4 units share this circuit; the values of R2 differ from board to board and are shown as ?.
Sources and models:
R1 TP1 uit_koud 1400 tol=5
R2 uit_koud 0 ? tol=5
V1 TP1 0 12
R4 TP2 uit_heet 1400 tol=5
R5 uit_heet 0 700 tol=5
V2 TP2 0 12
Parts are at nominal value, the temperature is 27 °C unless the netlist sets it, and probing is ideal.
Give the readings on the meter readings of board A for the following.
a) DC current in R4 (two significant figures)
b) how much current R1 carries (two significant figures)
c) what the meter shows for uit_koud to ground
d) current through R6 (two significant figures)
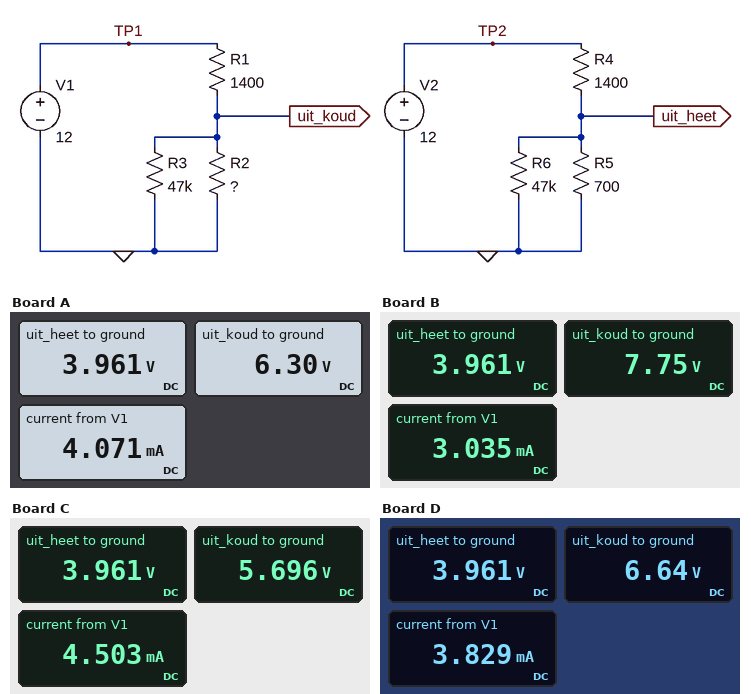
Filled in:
5.7 mA
4.1 mA
6.30 V
84 µA
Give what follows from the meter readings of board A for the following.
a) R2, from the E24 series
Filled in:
1.6 kΩ
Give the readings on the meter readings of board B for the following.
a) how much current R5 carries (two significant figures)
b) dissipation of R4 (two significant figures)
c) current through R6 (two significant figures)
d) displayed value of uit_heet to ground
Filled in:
5.7 mA
46 mW
84 µA
3.961 V
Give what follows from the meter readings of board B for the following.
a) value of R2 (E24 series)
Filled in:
2.7 kΩ
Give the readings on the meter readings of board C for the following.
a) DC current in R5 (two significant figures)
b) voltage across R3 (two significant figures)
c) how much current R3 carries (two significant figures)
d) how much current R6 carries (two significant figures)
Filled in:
5.7 mA
5.7 V
120 µA
84 µA
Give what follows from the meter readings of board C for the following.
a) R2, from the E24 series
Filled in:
1.3 kΩ
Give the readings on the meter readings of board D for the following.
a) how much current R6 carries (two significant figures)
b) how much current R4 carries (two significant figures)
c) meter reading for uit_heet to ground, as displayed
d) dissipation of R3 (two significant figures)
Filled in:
84 µA
5.7 mA
3.961 V
940 µW
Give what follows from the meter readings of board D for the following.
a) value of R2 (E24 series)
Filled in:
1.8 kΩ
